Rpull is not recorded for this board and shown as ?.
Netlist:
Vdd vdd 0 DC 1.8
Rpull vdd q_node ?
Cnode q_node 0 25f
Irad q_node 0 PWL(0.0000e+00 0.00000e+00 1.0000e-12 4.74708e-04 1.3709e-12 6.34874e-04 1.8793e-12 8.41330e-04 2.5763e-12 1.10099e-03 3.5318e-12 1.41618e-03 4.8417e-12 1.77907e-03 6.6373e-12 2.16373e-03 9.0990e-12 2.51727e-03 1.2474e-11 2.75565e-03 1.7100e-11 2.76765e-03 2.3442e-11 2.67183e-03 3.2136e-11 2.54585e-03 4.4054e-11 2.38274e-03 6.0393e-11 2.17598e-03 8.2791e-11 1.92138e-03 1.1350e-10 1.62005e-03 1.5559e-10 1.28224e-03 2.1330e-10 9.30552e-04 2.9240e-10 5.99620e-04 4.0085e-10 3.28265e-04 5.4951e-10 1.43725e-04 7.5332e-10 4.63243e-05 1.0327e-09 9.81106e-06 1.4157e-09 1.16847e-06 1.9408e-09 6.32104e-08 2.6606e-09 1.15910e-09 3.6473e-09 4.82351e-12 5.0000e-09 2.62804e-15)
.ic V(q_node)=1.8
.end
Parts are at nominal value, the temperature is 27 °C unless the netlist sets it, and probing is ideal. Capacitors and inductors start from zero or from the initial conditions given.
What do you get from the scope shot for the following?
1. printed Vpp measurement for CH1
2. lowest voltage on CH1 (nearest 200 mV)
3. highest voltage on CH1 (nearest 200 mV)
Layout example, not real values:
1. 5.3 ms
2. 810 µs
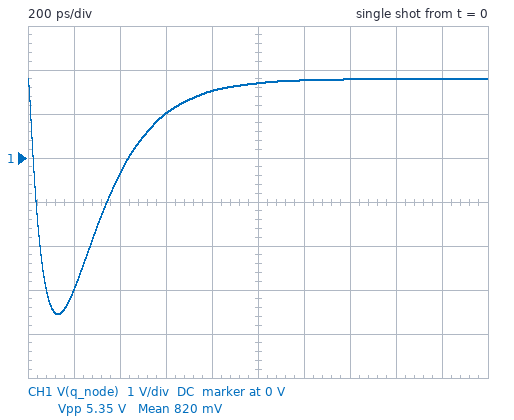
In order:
1. 5.35 V
2. -3.6 V
3. 1.8 V
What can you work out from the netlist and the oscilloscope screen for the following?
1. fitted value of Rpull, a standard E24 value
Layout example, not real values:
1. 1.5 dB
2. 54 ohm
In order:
1. 3.6 kΩ
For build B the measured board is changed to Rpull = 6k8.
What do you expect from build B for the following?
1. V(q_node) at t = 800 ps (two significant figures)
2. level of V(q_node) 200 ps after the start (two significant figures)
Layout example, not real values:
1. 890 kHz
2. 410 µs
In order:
1. 750 mV
2. -5.8 V
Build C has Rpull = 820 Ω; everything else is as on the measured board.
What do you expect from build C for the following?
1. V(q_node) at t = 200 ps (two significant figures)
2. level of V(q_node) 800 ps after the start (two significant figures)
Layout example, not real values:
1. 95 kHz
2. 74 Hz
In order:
1. 860 mV
2. 1.8 V
